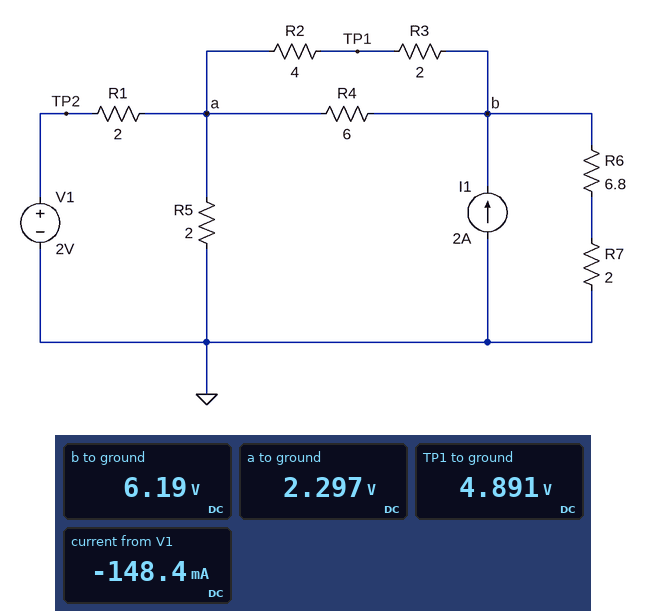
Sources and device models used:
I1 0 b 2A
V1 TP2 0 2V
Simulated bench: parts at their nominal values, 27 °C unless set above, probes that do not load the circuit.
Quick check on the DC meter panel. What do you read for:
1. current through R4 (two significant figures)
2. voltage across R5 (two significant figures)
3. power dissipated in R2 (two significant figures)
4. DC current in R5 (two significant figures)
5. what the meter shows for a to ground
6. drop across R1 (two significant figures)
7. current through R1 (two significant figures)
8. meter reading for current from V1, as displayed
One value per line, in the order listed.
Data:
650 mA
2.3 V
1.7 W
1.1 A
2.297 V
300 mV
150 mA
-148.4 mA
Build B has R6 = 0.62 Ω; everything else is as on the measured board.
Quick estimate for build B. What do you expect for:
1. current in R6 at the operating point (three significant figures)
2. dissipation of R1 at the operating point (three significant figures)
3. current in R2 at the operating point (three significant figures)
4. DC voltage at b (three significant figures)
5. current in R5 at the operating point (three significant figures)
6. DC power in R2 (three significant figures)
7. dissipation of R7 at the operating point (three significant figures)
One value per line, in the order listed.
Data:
1.36 A
64.6 mW
320 mA
3.56 V
820 mA
410 mW
3.70 W
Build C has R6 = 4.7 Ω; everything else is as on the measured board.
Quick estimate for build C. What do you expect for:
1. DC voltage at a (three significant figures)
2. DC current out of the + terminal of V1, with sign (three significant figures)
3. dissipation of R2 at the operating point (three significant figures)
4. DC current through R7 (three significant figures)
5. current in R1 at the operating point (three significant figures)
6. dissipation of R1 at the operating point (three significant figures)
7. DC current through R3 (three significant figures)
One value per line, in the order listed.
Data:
2.16 V
-79.4 mA
1.34 W
841 mA
79.4 mA
12.6 mW
579 mA
